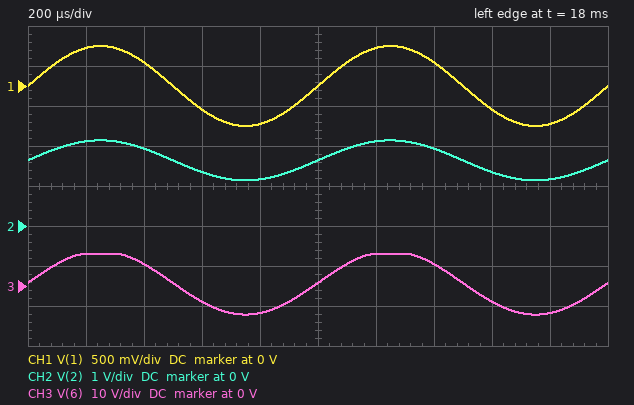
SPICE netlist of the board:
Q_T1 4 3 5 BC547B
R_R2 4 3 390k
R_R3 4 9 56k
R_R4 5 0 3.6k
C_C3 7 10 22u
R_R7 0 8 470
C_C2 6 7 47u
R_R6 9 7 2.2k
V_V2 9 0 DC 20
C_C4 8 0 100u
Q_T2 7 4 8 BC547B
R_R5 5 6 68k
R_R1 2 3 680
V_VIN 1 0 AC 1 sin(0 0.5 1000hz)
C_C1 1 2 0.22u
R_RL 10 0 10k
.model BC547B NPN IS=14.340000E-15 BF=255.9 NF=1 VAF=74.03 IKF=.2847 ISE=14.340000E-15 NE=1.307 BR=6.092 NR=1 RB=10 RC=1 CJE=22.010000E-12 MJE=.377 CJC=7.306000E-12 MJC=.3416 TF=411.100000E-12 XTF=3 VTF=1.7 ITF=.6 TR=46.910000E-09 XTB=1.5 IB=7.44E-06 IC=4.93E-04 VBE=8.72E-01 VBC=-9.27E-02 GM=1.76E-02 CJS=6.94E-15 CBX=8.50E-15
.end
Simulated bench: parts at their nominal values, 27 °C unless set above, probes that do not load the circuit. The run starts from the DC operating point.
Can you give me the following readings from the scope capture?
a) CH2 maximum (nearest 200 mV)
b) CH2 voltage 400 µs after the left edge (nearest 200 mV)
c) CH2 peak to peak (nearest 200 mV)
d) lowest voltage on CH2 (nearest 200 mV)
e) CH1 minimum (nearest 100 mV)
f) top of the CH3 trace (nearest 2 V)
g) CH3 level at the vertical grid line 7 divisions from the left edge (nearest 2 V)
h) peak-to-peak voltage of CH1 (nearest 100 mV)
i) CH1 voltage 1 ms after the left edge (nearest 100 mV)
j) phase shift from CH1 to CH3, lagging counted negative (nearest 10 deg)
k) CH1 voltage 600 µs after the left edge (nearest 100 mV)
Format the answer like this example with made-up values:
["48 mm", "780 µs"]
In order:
["2.2 V", "2.0 V", "1.0 V", "1.2 V", "-500 mV", "8 V", "6 V", "1.0 V", "0 V", "0 deg", "-300 mV"]
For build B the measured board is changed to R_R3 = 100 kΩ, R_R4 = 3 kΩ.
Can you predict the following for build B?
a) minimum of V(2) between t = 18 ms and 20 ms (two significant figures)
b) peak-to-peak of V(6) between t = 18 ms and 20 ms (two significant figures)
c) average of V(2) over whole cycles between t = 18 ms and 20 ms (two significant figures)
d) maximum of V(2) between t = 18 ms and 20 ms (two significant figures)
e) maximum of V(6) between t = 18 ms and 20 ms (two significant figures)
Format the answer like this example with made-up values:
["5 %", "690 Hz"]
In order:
["390 mV", "17 V", "890 mV", "1.4 V", "4.2 V"]
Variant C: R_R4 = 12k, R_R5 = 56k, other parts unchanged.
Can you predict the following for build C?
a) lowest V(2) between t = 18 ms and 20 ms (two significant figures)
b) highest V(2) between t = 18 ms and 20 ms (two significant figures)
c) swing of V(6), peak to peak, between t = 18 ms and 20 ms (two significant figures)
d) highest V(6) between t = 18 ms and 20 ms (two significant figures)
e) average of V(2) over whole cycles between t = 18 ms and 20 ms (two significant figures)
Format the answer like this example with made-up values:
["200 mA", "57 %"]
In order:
["3.0 V", "4.0 V", "2.4 V", "5.1 V", "3.5 V"]
